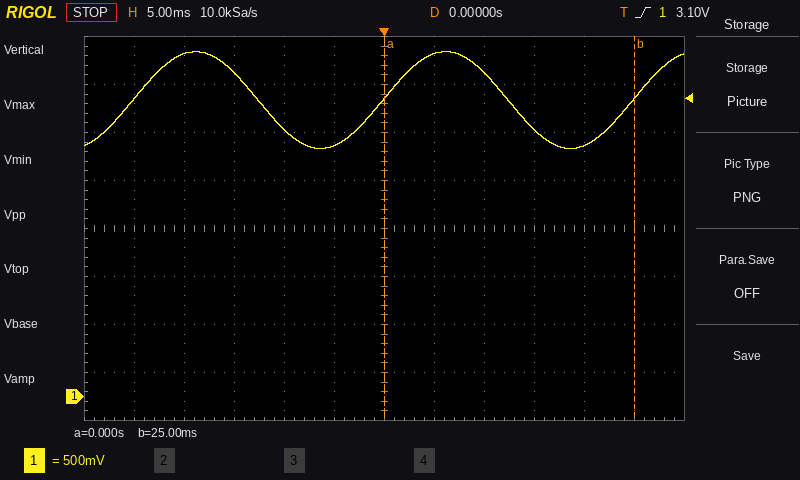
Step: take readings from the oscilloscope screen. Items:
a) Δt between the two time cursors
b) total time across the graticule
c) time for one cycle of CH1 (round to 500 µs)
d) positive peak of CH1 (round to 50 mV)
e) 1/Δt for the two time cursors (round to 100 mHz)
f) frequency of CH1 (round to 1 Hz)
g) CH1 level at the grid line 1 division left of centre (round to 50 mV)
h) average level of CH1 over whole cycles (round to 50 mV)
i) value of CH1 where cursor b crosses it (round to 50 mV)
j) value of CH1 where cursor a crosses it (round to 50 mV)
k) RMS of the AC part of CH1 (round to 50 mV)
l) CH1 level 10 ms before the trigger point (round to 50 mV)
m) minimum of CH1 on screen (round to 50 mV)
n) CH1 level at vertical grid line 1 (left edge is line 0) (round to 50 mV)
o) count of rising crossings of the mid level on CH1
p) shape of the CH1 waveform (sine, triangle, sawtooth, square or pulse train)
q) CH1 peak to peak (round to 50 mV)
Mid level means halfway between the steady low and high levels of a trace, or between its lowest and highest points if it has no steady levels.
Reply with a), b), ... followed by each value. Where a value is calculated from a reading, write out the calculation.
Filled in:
a) 25 ms − (0 s) = 25.0 ms
b) 60 ms
c) 25.0 ms
d) 3.60 V
e) 1 / 25.0 ms ≈ 40.0 Hz
f) 1 / 25.0 ms ≈ 40 Hz
g) 2.60 V
h) (3.60 V + (2.60 V)) / 2 ≈ 3.10 V
i) 3.10 V
j) 3.10 V
k) 1.00 V / (2√2) ≈ 354 mV, so 350 mV to the nearest 50 mV
l) 2.80 V
m) 2.60 V
n) 3.10 V
o) 3
p) sine
q) 3.60 V − (2.60 V) = 1.00 V
